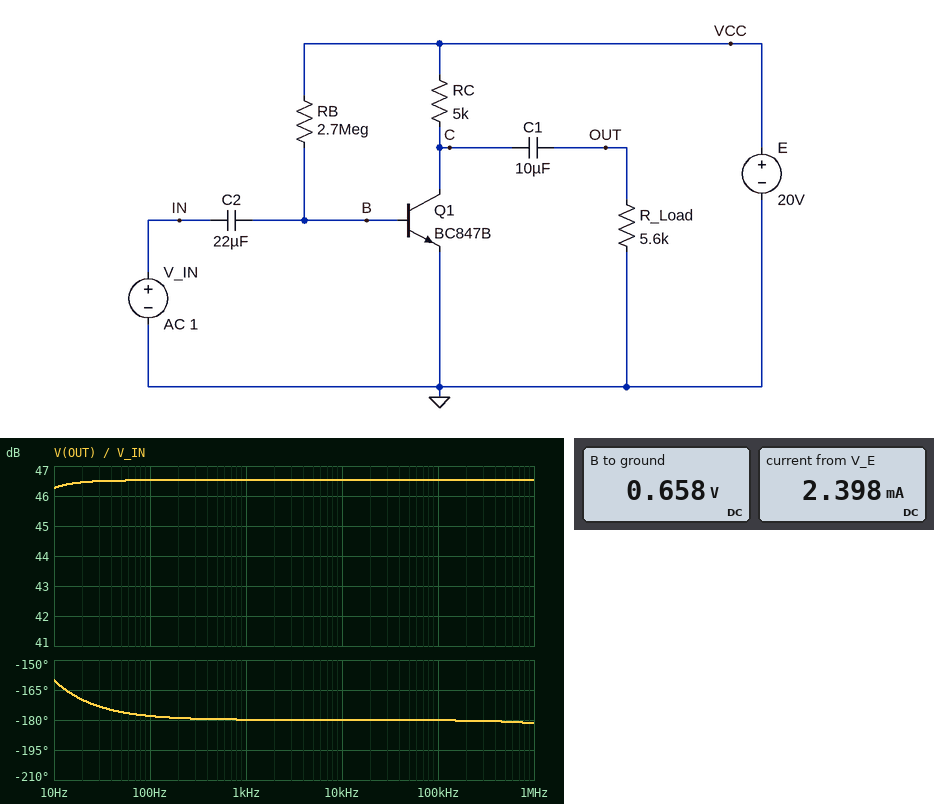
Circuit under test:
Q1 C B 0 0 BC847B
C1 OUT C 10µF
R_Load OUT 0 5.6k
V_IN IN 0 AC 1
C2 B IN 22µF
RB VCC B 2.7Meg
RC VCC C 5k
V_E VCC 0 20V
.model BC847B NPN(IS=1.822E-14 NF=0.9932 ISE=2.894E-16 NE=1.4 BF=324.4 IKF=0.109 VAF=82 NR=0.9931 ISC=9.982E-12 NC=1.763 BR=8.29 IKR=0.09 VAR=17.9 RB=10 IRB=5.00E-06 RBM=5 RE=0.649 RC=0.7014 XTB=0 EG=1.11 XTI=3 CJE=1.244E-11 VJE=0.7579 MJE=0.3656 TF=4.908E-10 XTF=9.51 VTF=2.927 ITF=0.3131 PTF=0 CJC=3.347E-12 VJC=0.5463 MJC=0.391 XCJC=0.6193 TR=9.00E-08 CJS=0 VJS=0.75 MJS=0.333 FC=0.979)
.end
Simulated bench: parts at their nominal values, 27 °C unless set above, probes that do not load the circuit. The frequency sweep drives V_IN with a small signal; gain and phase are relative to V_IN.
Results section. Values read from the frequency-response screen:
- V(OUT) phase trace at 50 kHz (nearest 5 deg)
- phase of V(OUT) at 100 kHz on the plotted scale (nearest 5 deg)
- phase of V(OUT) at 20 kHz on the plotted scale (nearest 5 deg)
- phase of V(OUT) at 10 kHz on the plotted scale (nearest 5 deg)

-180 deg
-180 deg
-180 deg
-180 deg
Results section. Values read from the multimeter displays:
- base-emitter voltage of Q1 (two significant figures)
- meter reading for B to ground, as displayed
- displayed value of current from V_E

660 mV
0.658 V
2.398 mA
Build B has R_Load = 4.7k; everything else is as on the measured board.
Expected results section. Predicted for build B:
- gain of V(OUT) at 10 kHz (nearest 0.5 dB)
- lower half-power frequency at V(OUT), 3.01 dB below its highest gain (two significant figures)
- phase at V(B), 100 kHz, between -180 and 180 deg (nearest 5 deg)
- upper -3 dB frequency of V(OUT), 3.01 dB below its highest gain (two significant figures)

46.0 dB
2.8 Hz
0 deg
41 MHz
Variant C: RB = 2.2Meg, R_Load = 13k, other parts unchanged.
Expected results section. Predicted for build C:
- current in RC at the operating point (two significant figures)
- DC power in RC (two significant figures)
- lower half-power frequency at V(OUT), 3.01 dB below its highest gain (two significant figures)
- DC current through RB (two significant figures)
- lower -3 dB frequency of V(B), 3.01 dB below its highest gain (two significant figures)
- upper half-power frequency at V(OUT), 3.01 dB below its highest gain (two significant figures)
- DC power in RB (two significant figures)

2.8 mA
40 mW
2.6 Hz
8.8 µA
2.3 Hz
25 MHz
170 µW
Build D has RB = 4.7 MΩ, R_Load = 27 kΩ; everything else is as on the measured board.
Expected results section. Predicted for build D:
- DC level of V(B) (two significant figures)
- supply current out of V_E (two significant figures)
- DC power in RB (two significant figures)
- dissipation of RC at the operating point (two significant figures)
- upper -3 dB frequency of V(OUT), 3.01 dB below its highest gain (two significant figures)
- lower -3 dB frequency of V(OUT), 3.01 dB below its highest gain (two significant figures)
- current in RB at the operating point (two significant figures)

640 mV
1.5 mA
80 µW
11 mW
32 MHz
1.3 Hz
4.1 µA
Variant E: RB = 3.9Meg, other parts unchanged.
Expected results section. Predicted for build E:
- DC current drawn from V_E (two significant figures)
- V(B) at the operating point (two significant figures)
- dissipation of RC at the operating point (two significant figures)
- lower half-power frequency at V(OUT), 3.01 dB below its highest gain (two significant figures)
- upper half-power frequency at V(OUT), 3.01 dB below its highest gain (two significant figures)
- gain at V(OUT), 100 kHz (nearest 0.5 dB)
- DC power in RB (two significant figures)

1.7 mA
650 mV
15 mW
2.3 Hz
46 MHz
44.0 dB
96 µW
